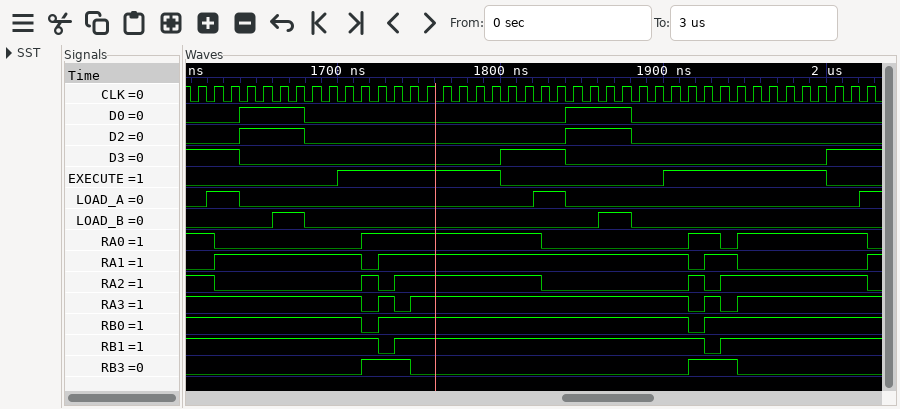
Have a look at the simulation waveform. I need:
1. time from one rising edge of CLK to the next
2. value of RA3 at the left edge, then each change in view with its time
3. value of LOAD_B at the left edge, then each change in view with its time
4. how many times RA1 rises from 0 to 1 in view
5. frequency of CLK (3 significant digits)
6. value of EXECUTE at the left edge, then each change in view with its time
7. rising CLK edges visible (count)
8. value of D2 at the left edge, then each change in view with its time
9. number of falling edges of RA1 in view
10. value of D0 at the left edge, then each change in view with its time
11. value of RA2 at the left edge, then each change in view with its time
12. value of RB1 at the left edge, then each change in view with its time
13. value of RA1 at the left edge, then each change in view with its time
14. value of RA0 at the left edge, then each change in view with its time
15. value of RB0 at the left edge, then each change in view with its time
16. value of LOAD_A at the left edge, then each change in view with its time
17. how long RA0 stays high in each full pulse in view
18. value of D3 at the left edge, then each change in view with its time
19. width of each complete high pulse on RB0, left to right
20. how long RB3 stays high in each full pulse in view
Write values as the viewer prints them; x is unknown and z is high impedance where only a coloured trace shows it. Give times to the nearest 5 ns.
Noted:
10 ns
1, 0 at 1715 ns, 1 at 1725 ns, 0 at 1735 ns, 1 at 1745 ns, 0 at 1915 ns, 1 at 1925 ns, 0 at 1935 ns, 1 at 1945 ns
0, 1 at 1660 ns, 0 at 1680 ns, 1 at 1860 ns, 0 at 1880 ns
4
100 MHz
0, 1 at 1700 ns, 0 at 1800 ns, 1 at 1900 ns, 0 at 2000 ns
42
0, 1 at 1640 ns, 0 at 1680 ns, 1 at 1840 ns, 0 at 1880 ns
3
0, 1 at 1640 ns, 0 at 1680 ns, 1 at 1840 ns, 0 at 1880 ns
1, 0 at 1625 ns, 1 at 1715 ns, 0 at 1725 ns, 1 at 1735 ns, 0 at 1825 ns, 1 at 1915 ns, 0 at 1925 ns, 1 at 1935 ns, 0 at 2025 ns
1, 0 at 1725 ns, 1 at 1735 ns, 0 at 1925 ns, 1 at 1935 ns
0, 1 at 1625 ns, 0 at 1715 ns, 1 at 1725 ns, 0 at 1915 ns, 1 at 1925 ns, 0 at 1945 ns, 1 at 2025 ns
1, 0 at 1625 ns, 1 at 1715 ns, 0 at 1825 ns, 1 at 1915 ns, 0 at 1935 ns, 1 at 1945 ns, 0 at 2025 ns
1, 0 at 1715 ns, 1 at 1725 ns, 0 at 1915 ns, 1 at 1925 ns
0, 1 at 1620 ns, 0 at 1640 ns, 1 at 1820 ns, 0 at 1840 ns, 1 at 2020 ns
110 ns, 20 ns, 80 ns
1, 0 at 1640 ns, 1 at 1800 ns, 0 at 1840 ns, 1 at 2000 ns
190 ns
30 ns, 30 ns
